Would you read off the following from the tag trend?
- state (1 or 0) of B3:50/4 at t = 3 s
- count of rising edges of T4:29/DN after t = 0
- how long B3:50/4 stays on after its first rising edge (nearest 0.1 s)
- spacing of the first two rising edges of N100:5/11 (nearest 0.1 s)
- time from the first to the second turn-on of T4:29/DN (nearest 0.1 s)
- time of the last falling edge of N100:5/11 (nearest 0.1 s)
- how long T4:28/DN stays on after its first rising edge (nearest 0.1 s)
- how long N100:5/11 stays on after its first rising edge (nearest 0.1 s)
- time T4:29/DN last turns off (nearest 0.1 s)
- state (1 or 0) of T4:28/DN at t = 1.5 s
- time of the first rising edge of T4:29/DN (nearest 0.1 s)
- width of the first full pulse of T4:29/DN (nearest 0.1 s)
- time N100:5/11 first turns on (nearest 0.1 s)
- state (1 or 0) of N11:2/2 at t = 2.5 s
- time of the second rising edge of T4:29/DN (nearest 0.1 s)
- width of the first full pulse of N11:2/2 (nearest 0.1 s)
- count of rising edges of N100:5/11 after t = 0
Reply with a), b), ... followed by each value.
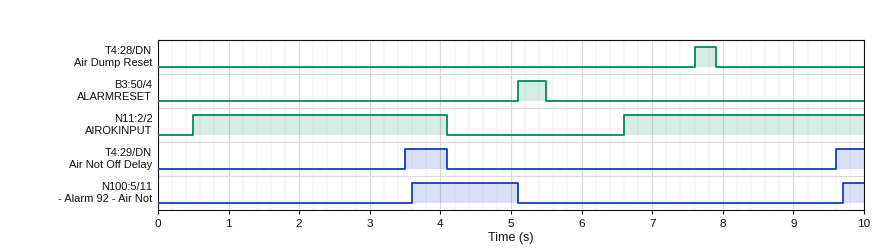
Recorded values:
a) 0
b) 2
c) 0.4 s
d) 6.1 s
e) 6.1 s
f) 5.1 s
g) 0.3 s
h) 1.5 s
i) 4.1 s
j) 0
k) 3.5 s
l) 0.6 s
m) 3.6 s
n) 1
o) 9.6 s
p) 3.6 s
q) 2
